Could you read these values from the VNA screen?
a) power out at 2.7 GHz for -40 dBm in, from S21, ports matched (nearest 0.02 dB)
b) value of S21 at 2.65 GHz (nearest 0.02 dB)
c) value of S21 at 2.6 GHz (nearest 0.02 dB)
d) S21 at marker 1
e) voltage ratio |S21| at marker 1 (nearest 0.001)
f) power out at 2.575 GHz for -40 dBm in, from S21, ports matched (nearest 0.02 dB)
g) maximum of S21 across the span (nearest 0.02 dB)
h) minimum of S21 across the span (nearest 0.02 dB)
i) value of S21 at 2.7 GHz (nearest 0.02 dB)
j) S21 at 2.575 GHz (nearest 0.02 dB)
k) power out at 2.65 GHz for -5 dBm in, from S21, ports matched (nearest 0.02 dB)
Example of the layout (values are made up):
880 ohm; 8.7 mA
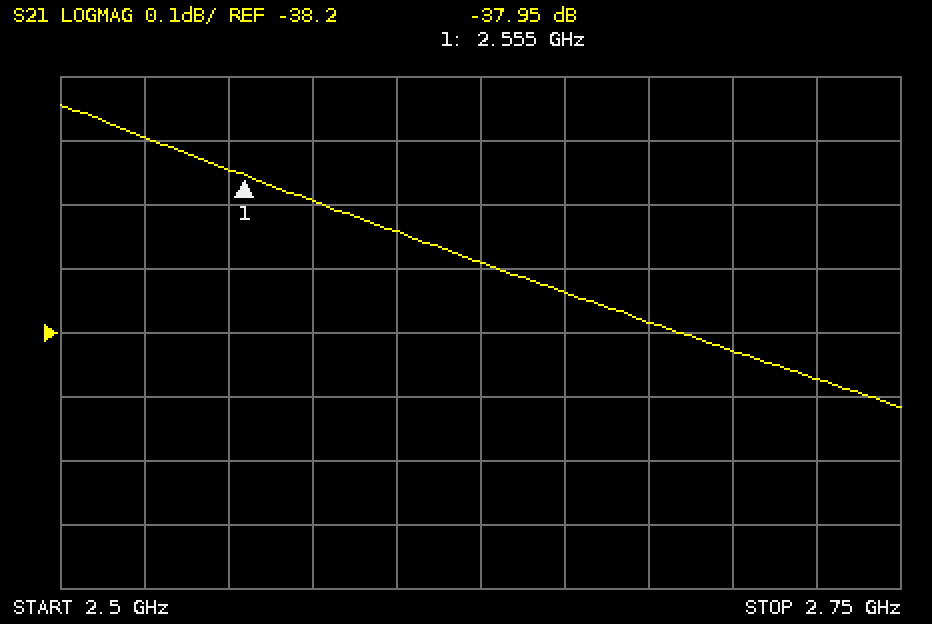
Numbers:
-78.22 dBm; -38.14 dB; -38.04 dB; -37.95 dB; 0.013; -78.00 dBm; -37.84 dB; -38.32 dB; -38.22 dB; -38.00 dB; -43.14 dBm
